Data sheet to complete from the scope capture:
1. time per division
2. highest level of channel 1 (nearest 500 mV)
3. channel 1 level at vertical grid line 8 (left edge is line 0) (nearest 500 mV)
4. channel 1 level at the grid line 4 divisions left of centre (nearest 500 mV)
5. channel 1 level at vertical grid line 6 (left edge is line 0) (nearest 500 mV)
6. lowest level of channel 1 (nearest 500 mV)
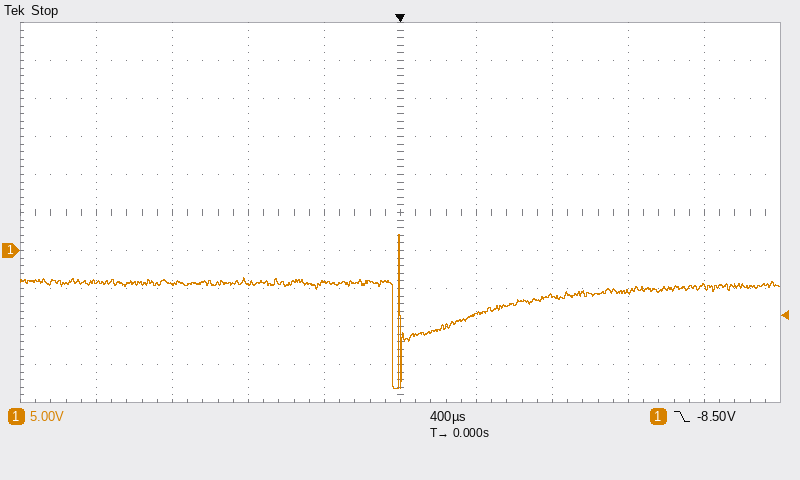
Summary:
400 µs
2.0 V
-5.5 V
-4.0 V
-8.5 V
-18.0 V
